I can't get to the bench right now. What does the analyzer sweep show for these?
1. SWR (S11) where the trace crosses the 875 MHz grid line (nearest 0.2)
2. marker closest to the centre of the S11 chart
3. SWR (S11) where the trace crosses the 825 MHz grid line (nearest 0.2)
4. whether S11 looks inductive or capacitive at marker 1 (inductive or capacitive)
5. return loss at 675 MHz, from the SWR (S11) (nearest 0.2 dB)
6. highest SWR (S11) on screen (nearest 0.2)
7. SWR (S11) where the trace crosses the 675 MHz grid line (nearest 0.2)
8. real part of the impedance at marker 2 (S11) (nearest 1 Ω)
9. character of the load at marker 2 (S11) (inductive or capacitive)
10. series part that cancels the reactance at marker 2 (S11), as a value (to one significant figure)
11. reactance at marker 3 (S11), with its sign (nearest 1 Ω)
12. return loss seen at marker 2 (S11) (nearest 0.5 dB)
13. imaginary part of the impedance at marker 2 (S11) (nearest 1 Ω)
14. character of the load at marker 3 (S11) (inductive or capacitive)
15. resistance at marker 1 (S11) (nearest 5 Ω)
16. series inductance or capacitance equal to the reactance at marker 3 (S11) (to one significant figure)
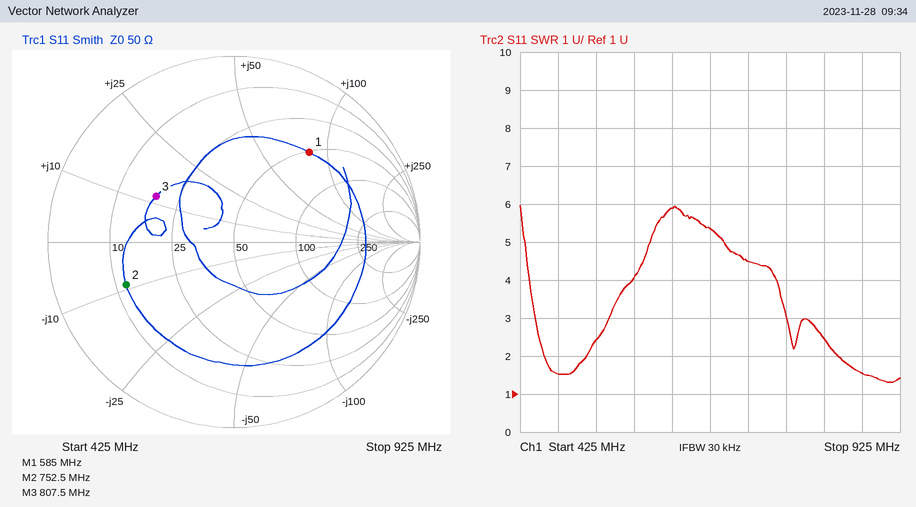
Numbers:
1.6
marker 3
2.4
inductive
3.2 dB
6.0
5.4
12 Ω
capacitive
2 nH
+12 Ω
4.0 dB
-9 Ω
inductive
50 Ω
2 nH
